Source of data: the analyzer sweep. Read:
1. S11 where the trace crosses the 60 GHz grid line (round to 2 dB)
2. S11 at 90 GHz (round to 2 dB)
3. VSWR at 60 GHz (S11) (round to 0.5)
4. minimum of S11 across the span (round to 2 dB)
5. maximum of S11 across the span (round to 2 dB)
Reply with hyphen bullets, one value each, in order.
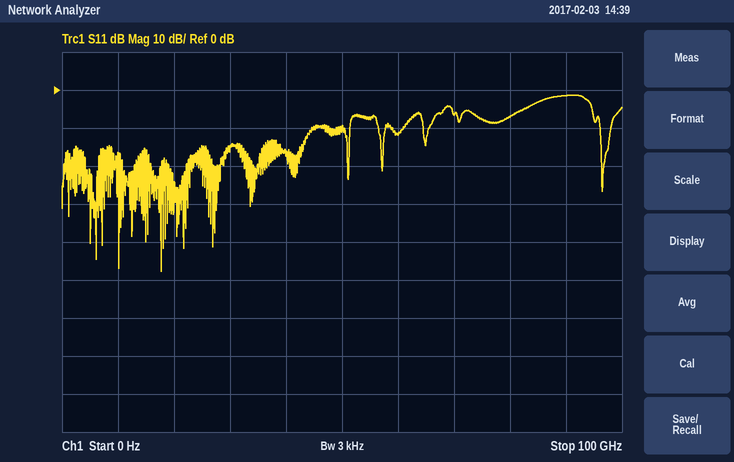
- -12 dB
- -2 dB
- 1.5
- -48 dB
- -2 dB
